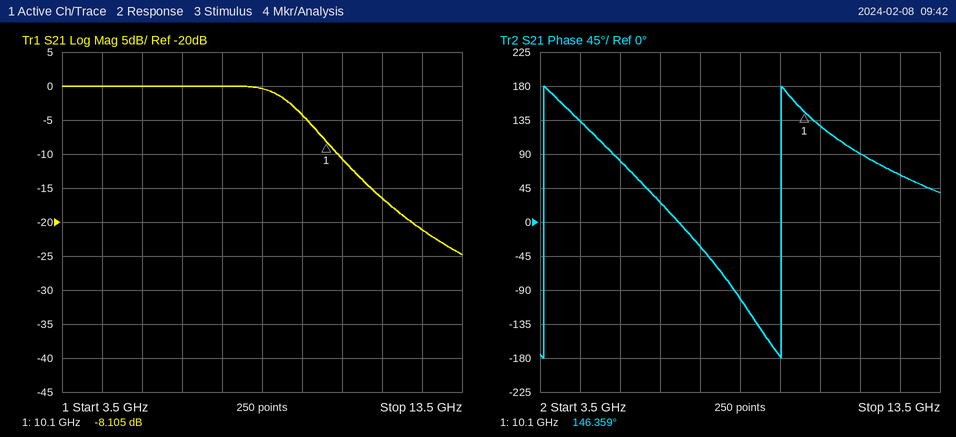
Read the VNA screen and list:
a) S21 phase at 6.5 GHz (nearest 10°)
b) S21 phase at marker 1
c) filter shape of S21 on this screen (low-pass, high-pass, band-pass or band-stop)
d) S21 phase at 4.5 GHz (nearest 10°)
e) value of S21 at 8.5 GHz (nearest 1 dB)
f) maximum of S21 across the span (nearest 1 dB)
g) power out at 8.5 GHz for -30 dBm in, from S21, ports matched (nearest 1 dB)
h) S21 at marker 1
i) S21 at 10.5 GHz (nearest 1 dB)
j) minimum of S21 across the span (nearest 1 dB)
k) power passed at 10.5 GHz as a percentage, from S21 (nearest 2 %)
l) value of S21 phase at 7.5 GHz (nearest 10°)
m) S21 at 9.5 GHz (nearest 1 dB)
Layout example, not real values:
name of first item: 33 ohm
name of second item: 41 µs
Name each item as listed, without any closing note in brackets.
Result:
S21 phase at 6.5 GHz: 30°
S21 phase at marker 1: 146.359°
filter shape of S21 on this screen: low-pass
S21 phase at 4.5 GHz: 130°
value of S21 at 8.5 GHz: 0 dB
maximum of S21 across the span: 0 dB
power out at 8.5 GHz for -30 dBm in, from S21, ports matched: -30 dBm
S21 at marker 1: -8.105 dB
S21 at 10.5 GHz: -11 dB
minimum of S21 across the span: -25 dB
power passed at 10.5 GHz as a percentage, from S21: 8 %
value of S21 phase at 7.5 GHz: -30°
S21 at 9.5 GHz: -4 dB
